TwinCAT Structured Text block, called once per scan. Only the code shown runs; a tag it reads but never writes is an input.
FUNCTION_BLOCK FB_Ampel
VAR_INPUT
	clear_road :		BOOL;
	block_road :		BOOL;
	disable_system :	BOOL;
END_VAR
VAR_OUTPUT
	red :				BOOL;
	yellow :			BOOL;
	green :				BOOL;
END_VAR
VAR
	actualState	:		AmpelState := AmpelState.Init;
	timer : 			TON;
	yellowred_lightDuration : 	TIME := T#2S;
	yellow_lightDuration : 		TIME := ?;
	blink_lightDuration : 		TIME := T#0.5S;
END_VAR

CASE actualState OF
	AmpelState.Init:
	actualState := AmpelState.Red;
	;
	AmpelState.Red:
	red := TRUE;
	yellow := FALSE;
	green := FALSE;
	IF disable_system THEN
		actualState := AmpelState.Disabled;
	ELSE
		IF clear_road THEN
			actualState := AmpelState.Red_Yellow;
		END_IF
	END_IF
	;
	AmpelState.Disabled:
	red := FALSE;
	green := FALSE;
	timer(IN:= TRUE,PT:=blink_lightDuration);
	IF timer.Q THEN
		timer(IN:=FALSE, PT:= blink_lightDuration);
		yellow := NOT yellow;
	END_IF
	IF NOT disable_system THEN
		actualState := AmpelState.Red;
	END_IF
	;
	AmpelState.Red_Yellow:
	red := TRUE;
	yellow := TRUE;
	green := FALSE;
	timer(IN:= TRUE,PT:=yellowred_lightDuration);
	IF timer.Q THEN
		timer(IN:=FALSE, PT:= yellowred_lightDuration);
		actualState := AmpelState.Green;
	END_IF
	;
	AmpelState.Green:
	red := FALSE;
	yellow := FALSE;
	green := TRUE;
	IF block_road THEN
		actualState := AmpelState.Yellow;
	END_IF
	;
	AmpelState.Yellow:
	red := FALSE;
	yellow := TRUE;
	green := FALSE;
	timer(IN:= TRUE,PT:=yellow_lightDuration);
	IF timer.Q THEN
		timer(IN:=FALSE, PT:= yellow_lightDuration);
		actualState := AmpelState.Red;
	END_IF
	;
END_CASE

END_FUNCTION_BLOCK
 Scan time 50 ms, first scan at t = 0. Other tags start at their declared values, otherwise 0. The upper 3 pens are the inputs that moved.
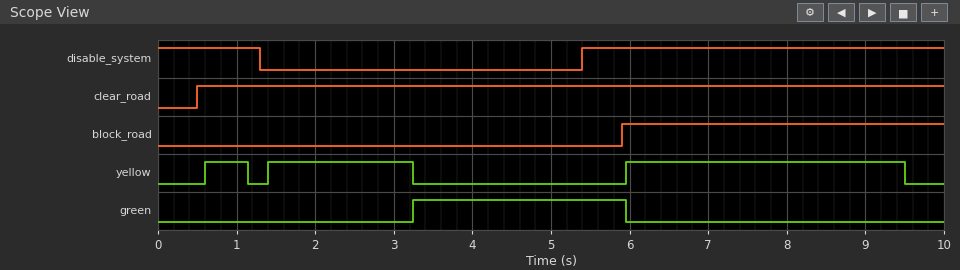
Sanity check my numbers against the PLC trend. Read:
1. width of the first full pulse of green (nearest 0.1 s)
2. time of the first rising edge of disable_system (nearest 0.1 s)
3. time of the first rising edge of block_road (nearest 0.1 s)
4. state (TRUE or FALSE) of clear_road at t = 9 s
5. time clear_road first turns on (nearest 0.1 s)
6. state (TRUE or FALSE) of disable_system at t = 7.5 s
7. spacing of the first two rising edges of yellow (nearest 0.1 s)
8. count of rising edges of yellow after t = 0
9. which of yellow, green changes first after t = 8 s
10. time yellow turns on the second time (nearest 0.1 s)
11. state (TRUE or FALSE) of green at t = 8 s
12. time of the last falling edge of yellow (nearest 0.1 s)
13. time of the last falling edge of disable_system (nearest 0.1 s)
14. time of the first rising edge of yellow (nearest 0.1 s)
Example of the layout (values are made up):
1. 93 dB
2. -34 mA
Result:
1. 2.7 s
2. 5.4 s
3. 5.9 s
4. TRUE
5. 0.5 s
6. TRUE
7. 0.8 s
8. 3
9. yellow
10. 1.4 s
11. FALSE
12. 9.5 s
13. 1.3 s
14. 0.6 s
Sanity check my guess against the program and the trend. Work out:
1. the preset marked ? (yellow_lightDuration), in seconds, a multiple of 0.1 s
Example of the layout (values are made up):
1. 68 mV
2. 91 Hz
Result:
1. 3.5 s
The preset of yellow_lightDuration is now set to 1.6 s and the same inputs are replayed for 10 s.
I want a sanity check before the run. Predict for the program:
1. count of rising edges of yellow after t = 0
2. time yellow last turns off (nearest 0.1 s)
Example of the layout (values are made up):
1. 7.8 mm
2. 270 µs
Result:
1. 5
2. 9.8 s
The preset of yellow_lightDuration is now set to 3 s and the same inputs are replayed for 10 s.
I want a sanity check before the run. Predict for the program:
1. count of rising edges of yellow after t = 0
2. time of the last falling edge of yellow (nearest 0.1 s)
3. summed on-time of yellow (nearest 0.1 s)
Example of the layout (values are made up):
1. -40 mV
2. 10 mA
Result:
1. 4
2. 9.0 s
3. 5.9 s
